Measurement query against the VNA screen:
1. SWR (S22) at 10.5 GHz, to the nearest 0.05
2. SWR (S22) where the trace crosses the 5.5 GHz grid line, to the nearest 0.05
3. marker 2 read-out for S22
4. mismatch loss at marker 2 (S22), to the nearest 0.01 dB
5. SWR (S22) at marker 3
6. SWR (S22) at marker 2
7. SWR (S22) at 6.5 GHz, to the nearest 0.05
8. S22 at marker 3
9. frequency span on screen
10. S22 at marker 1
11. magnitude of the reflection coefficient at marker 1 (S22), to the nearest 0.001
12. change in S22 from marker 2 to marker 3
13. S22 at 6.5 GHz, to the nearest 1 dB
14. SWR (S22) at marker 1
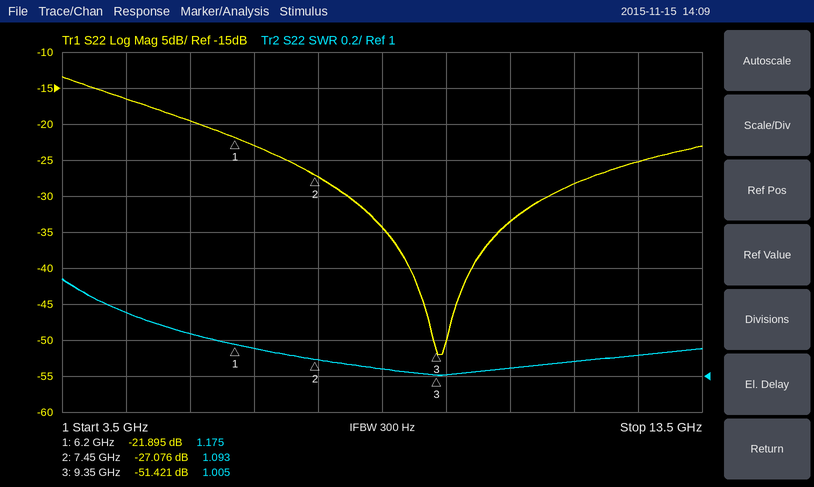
1.05
1.25
-27.076 dB
0.01 dB
1.005
1.093
1.15
-51.421 dB
10 GHz
-21.895 dB
0.080
-24.345 dB
-23 dB
1.175
